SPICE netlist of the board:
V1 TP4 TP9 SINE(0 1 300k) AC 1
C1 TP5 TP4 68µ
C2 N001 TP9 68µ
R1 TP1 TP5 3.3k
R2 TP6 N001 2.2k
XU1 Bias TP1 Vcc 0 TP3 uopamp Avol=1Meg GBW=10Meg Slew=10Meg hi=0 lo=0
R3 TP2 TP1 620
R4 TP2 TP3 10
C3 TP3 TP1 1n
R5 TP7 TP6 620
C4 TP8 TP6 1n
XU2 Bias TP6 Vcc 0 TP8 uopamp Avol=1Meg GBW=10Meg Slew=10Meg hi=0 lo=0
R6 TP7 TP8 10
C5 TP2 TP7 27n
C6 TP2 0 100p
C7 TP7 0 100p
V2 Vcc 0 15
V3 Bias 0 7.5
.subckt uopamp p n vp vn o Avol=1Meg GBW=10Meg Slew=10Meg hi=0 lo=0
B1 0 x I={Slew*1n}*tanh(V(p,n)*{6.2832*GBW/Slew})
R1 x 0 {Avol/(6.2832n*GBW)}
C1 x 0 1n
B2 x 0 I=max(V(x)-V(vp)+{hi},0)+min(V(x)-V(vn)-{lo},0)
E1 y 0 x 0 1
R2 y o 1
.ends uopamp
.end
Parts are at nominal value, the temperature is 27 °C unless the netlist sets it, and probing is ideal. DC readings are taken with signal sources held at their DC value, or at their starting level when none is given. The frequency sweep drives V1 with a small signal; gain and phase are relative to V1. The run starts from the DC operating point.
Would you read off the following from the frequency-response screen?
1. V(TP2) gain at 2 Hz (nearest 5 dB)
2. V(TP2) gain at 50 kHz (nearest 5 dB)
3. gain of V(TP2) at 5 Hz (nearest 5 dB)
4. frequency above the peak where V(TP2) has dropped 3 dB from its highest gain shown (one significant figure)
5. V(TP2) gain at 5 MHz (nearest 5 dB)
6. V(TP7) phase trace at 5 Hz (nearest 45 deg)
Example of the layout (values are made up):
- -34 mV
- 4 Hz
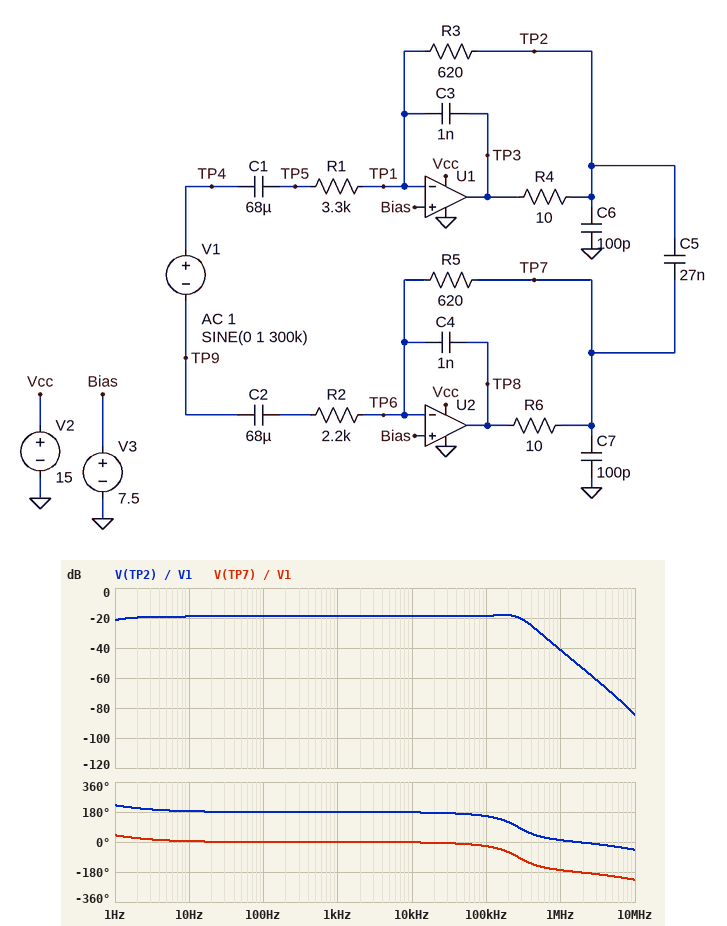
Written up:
- -20 dB
- -20 dB
- -20 dB
- 300 kHz
- -70 dB
- 0 deg
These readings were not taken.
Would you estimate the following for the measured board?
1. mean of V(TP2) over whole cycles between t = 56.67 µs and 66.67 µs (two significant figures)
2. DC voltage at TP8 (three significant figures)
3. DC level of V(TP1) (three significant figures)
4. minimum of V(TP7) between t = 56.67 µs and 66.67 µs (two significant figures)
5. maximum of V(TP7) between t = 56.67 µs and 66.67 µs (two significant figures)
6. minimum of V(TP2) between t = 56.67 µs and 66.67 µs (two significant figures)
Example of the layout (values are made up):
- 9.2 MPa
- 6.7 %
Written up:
- 7.5 V
- 7.50 V
- 7.50 V
- 7.4 V
- 7.6 V
- 7.4 V
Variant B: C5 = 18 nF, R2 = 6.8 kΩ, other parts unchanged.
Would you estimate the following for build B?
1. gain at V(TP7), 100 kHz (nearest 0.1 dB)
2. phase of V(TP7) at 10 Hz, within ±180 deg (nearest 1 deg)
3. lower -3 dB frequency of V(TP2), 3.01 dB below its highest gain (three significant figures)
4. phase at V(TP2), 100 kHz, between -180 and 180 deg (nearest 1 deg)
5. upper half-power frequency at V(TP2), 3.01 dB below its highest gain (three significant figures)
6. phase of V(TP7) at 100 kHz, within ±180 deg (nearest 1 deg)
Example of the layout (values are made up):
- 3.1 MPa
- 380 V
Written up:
- -24.2 dB
- 3 deg
- 472 mHz
- 156 deg
- 352 kHz
- -24 deg
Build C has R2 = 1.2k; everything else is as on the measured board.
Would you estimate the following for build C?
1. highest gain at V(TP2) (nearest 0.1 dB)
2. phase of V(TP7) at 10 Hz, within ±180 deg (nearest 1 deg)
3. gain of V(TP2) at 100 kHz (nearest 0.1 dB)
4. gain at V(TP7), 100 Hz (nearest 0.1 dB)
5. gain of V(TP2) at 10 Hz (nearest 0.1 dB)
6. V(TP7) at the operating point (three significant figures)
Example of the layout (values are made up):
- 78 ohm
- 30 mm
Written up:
- -16.4 dB
- 6 deg
- -16.8 dB
- -17.2 dB
- -17.3 dB
- 7.50 V
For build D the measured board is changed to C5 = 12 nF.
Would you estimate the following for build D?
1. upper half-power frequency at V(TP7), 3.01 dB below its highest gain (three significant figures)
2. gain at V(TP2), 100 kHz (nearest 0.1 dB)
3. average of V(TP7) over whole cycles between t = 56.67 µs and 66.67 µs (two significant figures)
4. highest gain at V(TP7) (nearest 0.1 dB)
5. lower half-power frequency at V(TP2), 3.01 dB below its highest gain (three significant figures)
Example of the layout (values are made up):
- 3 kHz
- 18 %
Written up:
- 350 kHz
- -19.1 dB
- 7.5 V
- -19.0 dB
- 851 mHz
